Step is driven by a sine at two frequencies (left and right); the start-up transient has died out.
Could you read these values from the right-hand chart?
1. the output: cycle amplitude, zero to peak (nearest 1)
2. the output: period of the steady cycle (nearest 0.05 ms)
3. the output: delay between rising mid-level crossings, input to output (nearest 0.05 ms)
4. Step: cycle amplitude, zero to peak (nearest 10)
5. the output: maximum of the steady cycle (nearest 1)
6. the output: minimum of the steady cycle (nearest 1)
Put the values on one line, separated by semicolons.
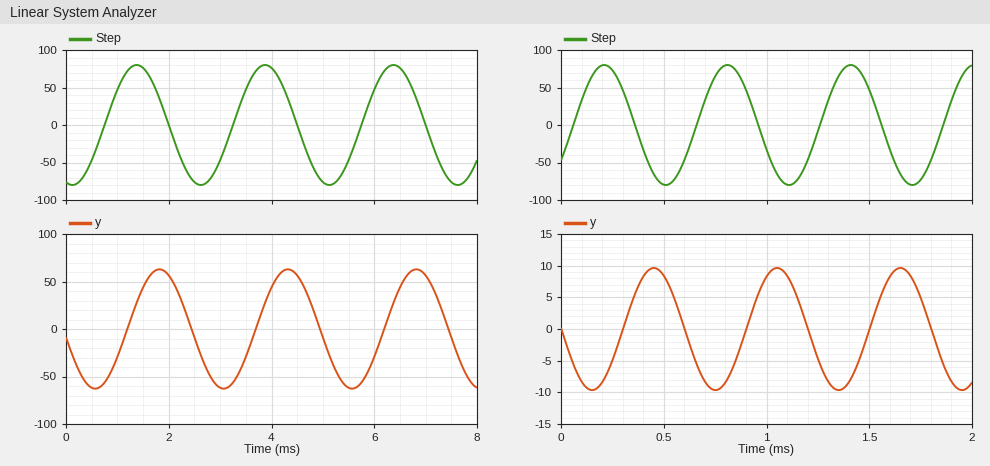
10; 0.60 ms; 0.25 ms; 80; 10; -10
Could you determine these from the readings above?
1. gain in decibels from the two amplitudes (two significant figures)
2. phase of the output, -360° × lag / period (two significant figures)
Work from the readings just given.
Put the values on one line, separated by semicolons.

-18 dB; -150°
